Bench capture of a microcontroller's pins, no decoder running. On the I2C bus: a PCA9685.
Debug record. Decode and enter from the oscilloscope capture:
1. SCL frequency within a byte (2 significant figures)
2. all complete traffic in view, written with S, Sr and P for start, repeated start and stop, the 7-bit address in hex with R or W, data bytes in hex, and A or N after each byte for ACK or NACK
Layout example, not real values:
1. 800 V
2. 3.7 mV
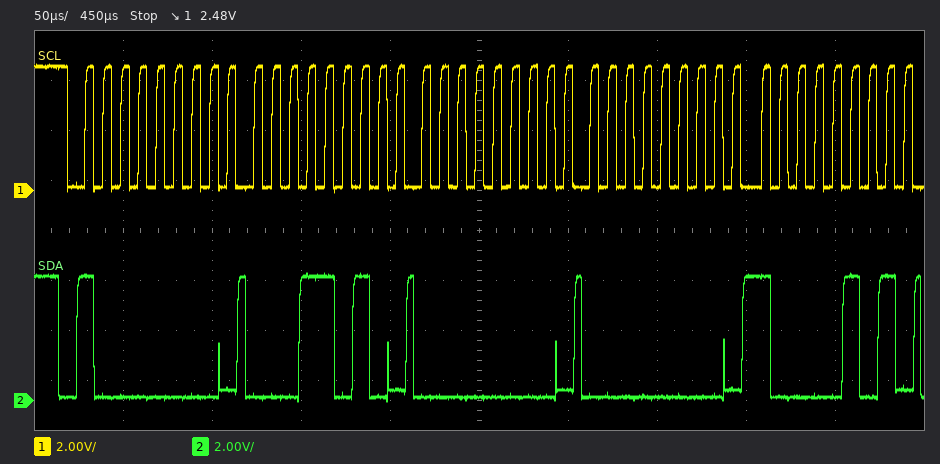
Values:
1. 100 kHz
2. S 40W A 1A A 00 A 00 A 85 A
